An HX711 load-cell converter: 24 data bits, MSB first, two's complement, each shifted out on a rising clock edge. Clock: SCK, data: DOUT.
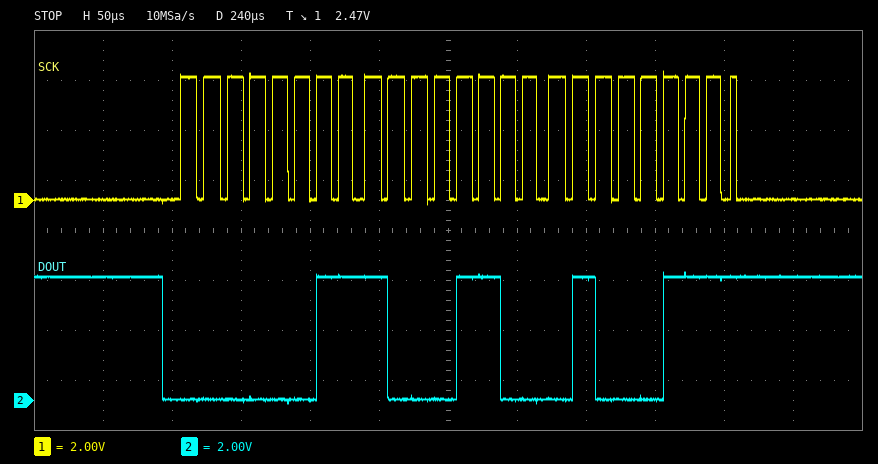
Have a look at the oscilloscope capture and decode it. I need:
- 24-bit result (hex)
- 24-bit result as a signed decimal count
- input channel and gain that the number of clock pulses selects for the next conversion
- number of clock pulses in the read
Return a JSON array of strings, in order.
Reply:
["0x038C47", "232519", "channel A, gain 128", "25"]
